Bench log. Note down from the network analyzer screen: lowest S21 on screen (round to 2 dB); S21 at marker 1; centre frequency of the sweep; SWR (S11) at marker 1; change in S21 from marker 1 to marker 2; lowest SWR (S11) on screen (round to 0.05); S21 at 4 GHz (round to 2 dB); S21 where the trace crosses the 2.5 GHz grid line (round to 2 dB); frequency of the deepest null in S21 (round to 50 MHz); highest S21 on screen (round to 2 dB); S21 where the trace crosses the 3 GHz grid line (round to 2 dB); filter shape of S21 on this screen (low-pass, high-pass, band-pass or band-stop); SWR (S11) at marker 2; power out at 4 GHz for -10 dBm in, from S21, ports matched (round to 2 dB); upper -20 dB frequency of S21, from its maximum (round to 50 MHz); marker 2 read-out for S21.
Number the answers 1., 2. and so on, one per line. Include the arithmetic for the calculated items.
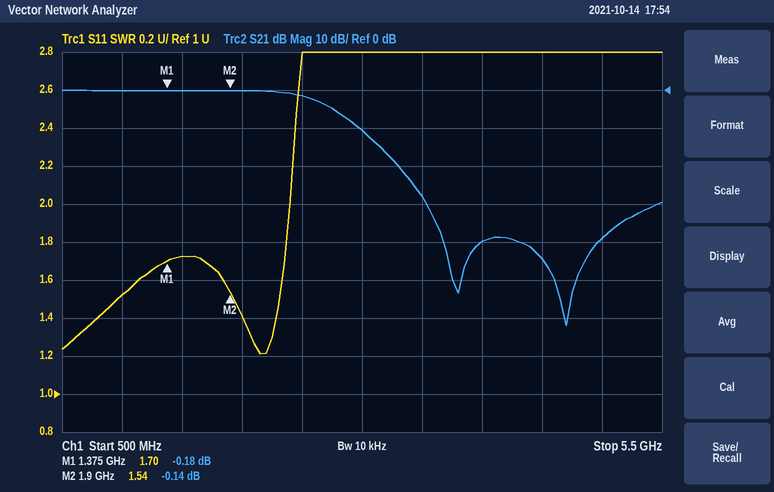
1. -62 dB
2. -0.18 dB
3. 3 GHz
4. 1.70
5. -0.14 − (-0.18) = 0.04 dB
6. 1.20
7. -40 dB
8. -2 dB
9. 4.70 GHz
10. 0 dB
11. -10 dB
12. low-pass
13. 1.54
14. -10 dBm + (-40 dB) = -50 dBm
15. 3.30 GHz
16. -0.14 dB
